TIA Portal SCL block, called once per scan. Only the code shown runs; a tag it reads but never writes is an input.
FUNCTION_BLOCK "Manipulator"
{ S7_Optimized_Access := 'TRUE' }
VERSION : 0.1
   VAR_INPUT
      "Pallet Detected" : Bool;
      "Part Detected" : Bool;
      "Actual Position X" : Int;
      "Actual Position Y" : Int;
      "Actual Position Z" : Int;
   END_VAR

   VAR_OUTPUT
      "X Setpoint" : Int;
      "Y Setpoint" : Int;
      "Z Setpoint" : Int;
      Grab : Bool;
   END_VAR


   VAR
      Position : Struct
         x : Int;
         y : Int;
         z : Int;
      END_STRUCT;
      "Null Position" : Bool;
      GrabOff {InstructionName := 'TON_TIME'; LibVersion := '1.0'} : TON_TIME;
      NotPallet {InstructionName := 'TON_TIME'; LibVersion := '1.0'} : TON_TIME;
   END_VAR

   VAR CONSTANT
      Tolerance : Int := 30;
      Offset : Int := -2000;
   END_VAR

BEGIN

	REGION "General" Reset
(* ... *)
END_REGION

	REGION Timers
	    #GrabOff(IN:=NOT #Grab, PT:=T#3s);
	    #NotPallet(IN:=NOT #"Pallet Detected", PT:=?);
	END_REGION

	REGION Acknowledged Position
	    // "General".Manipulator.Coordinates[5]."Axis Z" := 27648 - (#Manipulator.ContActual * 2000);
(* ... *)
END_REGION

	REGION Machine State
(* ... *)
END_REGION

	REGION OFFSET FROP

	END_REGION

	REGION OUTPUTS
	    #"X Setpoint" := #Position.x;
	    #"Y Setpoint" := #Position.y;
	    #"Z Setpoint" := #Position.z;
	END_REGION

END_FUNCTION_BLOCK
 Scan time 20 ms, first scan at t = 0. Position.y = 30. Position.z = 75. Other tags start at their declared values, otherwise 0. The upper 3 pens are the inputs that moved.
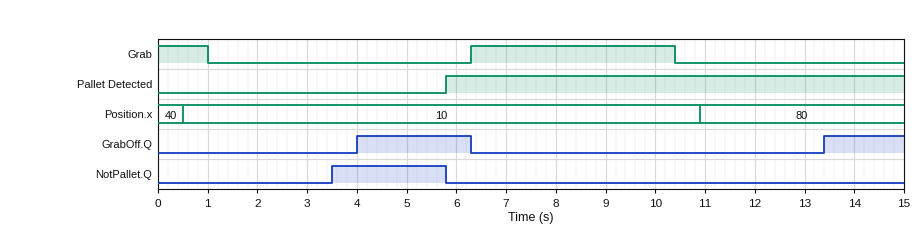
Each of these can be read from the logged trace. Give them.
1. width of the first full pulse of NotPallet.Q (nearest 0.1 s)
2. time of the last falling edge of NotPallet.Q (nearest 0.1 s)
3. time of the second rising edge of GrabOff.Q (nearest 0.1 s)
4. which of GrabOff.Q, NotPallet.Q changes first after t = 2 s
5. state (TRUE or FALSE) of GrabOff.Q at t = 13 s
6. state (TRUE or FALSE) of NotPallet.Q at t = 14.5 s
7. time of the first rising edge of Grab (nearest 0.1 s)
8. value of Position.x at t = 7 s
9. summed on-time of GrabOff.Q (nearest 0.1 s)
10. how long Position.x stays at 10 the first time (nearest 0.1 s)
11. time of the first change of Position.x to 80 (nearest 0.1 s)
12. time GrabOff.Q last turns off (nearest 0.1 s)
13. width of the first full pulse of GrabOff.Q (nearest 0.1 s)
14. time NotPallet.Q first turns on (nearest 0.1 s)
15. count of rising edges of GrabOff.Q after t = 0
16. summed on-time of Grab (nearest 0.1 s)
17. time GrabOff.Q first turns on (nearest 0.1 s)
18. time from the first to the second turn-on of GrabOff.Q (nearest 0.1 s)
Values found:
2.3 s
5.8 s
13.4 s
NotPallet.Q
FALSE
FALSE
6.3 s
10
3.9 s
10.4 s
10.9 s
6.3 s
2.3 s
3.5 s
2
5.1 s
4.0 s
9.4 s
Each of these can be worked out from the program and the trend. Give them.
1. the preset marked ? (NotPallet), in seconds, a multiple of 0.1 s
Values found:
3.5 s
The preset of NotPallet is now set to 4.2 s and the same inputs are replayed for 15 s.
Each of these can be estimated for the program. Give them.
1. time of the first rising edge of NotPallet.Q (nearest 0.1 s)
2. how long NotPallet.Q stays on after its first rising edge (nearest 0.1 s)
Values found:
4.2 s
1.6 s
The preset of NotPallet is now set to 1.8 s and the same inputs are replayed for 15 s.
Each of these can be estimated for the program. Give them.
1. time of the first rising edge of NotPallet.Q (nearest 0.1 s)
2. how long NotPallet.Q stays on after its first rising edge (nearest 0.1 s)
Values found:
1.8 s
4.0 s
